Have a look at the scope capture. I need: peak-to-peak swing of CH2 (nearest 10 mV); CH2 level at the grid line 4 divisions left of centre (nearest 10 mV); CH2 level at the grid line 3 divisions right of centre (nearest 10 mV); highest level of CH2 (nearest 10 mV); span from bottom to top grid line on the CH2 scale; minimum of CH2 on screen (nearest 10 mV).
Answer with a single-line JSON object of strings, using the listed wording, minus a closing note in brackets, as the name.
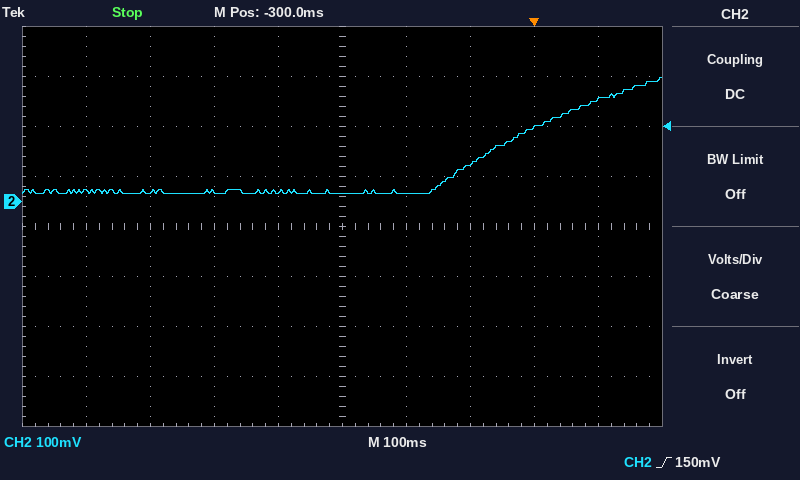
{"peak-to-peak swing of CH2": "230 mV", "CH2 level at the grid line 4 divisions left of centre": "20 mV", "CH2 level at the grid line 3 divisions right of centre": "150 mV", "highest level of CH2": "250 mV", "span from bottom to top grid line on the CH2 scale": "800 mV", "minimum of CH2 on screen": "20 mV"}
